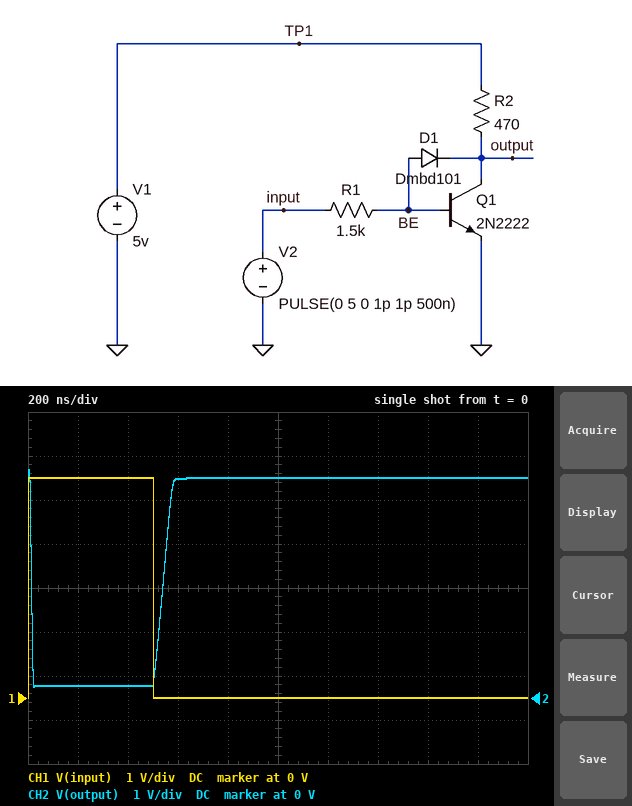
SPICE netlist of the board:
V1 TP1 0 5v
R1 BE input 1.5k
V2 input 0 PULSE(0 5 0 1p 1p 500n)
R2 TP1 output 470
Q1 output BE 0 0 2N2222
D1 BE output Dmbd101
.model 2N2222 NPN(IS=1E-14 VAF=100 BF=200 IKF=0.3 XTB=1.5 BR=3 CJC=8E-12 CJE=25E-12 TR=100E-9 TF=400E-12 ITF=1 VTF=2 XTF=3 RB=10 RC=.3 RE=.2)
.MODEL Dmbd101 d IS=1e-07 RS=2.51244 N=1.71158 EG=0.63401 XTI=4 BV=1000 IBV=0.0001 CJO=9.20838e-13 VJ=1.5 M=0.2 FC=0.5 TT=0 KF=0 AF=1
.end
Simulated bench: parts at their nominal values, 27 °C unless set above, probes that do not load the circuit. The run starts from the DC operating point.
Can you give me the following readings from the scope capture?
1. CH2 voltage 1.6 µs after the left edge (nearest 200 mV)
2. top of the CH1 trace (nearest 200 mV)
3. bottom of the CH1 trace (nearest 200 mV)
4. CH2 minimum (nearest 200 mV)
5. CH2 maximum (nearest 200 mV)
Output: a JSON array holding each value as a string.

["5.0 V", "5.0 V", "0 V", "200 mV", "5.2 V"]
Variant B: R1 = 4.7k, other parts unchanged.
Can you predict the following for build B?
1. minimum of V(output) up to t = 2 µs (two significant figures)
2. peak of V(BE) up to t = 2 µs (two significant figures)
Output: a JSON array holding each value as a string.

["320 mV", "730 mV"]
